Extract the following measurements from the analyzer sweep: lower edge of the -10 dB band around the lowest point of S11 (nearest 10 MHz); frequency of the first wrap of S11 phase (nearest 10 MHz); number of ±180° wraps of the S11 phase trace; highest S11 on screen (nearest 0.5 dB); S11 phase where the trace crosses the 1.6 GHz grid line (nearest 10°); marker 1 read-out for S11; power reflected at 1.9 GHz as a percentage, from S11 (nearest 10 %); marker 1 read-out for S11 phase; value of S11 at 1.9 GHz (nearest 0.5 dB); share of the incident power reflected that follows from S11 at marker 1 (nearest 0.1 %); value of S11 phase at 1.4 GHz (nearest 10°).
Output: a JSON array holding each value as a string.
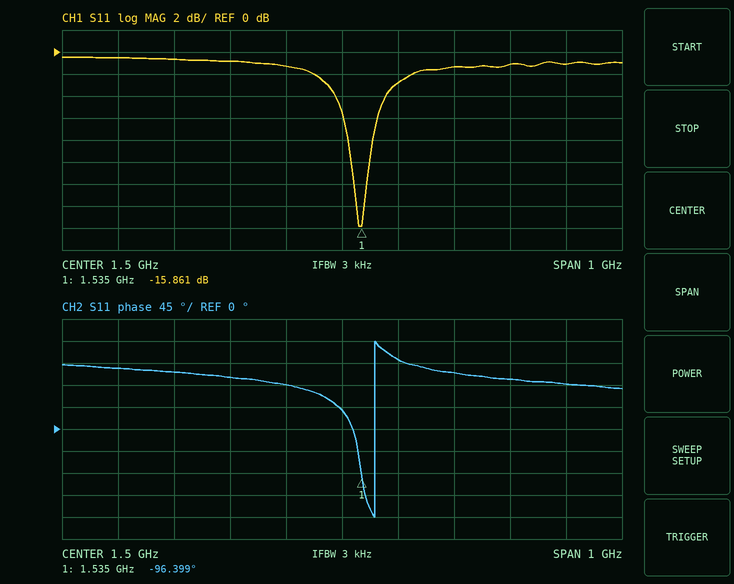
["1.52 GHz", "1.56 GHz", "1", "-0.5 dB", "140°", "-15.861 dB", "80 %", "-96.399°", "-1.0 dB", "2.6 %", "90°"]
